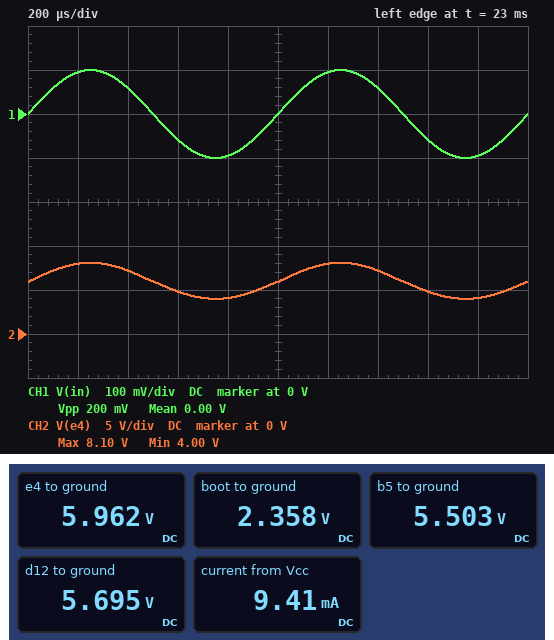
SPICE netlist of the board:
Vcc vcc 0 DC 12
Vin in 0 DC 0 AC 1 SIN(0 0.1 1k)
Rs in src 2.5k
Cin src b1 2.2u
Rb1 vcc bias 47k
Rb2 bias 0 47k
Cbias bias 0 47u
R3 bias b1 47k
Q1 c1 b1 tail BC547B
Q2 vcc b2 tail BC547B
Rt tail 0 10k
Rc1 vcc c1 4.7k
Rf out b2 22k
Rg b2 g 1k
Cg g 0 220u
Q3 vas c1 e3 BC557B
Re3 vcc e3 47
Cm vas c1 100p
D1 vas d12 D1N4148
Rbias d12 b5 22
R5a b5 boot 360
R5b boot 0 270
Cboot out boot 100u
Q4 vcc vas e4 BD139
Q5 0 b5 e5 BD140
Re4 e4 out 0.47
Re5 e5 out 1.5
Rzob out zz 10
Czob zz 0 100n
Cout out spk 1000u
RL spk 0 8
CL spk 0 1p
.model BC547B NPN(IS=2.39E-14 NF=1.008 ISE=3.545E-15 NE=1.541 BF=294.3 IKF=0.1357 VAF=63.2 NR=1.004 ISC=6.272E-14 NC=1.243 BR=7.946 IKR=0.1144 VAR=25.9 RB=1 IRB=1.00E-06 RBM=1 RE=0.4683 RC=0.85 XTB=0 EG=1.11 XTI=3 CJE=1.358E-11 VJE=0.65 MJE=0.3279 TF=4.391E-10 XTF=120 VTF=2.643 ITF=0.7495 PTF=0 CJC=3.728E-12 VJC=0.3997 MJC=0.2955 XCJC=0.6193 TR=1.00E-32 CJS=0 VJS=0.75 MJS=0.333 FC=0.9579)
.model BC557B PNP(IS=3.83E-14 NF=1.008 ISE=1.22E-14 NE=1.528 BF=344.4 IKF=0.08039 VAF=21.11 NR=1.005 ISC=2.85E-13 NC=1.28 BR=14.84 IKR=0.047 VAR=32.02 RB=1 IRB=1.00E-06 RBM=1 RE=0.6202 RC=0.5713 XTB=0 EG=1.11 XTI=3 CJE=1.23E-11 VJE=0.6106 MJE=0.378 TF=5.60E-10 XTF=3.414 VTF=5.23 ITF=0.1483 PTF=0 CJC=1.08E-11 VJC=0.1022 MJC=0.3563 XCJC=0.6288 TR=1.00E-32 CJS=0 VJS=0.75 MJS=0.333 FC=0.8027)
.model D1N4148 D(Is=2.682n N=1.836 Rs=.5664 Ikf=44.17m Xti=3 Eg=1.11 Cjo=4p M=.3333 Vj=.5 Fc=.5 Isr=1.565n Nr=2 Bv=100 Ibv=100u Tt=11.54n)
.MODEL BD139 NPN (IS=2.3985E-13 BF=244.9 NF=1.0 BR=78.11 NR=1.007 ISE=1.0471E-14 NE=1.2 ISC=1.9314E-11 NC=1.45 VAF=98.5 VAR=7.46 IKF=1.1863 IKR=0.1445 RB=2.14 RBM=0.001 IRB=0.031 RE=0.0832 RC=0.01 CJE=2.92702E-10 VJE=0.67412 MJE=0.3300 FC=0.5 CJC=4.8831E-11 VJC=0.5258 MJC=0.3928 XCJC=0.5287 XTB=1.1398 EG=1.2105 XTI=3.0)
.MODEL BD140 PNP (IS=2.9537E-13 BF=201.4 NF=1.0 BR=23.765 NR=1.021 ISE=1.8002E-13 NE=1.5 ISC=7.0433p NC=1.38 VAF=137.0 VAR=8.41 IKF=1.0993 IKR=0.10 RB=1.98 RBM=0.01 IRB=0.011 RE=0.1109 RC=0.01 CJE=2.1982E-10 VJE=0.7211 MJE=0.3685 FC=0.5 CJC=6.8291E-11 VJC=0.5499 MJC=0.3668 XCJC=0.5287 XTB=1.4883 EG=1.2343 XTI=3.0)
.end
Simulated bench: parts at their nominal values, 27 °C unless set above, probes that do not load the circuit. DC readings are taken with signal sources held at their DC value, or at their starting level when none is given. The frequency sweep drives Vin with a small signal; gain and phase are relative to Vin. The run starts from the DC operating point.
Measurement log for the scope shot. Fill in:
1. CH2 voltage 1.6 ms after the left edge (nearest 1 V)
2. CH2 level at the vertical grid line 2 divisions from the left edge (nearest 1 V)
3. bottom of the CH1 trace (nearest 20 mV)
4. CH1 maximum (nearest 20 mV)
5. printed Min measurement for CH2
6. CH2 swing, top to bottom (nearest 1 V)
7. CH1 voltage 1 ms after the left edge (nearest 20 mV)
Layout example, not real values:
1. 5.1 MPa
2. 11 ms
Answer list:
1. 5 V
2. 7 V
3. -100 mV
4. 100 mV
5. 4.00 V
6. 4 V
7. 0 V
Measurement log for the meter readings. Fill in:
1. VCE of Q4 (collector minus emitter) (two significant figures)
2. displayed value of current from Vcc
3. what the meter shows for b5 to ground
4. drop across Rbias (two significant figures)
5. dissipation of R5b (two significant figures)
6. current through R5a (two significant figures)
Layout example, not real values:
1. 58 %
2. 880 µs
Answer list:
1. 6.0 V
2. 9.41 mA
3. 5.503 V
4. 190 mV
5. 21 mW
6. 8.7 mA
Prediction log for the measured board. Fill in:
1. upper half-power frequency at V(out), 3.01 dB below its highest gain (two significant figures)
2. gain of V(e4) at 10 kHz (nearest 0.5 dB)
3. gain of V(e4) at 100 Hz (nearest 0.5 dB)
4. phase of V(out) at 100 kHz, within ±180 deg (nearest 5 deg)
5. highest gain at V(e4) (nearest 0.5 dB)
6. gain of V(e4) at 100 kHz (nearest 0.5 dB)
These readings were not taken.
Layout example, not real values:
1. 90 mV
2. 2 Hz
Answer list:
1. 8.2 Hz
2. 9.5 dB
3. 10.0 dB
4. -75 deg
5. 18.5 dB
6. 1.0 dB
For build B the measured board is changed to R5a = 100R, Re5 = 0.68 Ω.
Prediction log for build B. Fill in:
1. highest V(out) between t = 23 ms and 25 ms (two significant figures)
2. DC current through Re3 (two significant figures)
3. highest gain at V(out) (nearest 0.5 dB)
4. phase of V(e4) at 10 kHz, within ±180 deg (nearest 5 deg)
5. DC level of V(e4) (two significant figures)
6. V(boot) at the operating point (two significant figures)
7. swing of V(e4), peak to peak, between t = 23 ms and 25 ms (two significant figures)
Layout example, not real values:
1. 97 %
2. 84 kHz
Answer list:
1. 7.8 V
2. 15 mA
3. 25.0 dB
4. -5 deg
5. 5.9 V
6. 3.9 V
7. 3.8 V
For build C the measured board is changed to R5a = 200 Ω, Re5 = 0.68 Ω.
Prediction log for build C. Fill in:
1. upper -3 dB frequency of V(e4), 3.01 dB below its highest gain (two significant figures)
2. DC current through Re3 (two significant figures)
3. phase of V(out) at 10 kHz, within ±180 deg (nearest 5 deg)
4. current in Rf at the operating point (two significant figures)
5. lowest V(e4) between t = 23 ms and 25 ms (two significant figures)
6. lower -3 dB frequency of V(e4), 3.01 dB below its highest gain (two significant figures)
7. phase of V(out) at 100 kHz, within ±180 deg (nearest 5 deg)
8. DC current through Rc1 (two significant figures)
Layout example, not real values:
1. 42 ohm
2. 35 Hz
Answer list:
1. 8.5 Hz
2. 12 mA
3. -10 deg
4. 760 nA
5. 4.0 V
6. 1.2 Hz
7. -65 deg
8. 260 µA
